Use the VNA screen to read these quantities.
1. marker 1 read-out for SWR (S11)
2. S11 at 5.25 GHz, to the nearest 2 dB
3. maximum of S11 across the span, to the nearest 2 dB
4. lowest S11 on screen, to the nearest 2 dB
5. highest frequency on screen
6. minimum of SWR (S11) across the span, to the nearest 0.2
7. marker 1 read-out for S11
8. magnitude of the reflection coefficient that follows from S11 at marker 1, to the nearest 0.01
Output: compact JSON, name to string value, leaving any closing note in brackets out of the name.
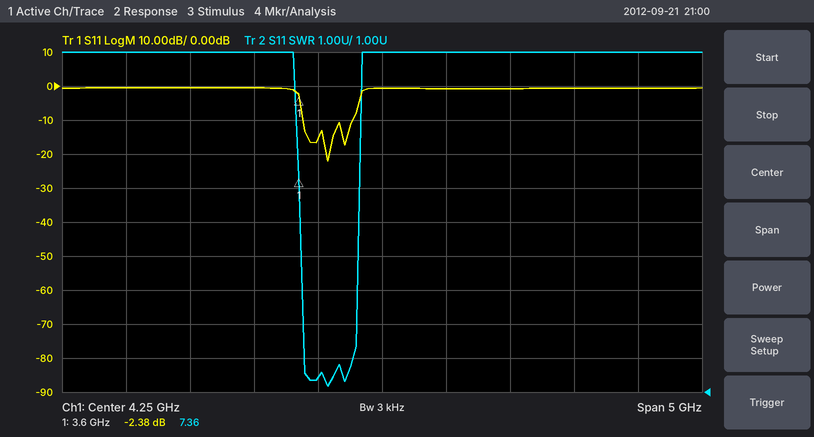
{"marker 1 read-out for SWR": "7.36", "S11 at 5.25 GHz, to the nearest 2 dB": "0 dB", "maximum of S11 across the span, to the nearest 2 dB": "0 dB", "lowest S11 on screen, to the nearest 2 dB": "-22 dB", "highest frequency on screen": "6.75 GHz", "minimum of SWR (S11) across the span, to the nearest 0.2": "1.2", "marker 1 read-out for S11": "-2.38 dB", "magnitude of the reflection coefficient that follows from S11 at marker 1, to the nearest 0.01": "0.76"}
